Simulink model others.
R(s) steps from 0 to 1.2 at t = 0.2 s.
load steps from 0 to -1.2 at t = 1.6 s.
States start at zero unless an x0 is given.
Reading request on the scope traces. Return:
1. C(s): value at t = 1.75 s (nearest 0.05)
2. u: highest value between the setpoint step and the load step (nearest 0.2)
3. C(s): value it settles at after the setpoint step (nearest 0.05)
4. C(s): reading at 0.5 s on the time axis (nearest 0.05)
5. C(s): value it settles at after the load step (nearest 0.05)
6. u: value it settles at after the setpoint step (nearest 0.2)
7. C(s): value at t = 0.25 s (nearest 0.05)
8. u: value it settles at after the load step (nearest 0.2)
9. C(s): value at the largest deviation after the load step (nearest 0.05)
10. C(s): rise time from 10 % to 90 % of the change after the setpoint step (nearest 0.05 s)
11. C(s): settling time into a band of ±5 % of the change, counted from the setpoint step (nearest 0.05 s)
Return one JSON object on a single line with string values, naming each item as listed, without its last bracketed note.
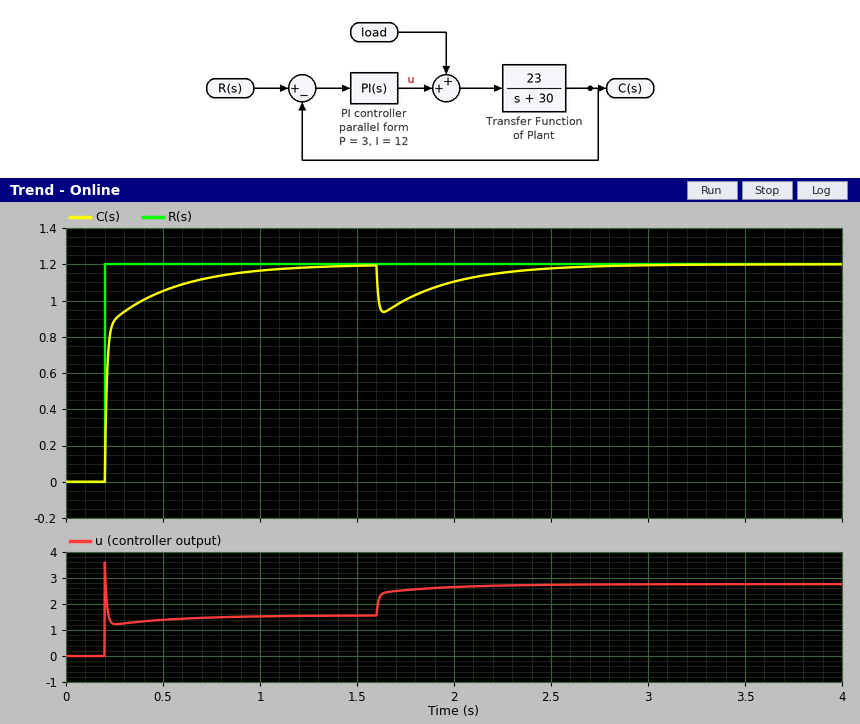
{"C(s): value at t = 1.75 s": "1.00", "u: highest value between the setpoint step and the load step": "3.6", "C(s): value it settles at after the setpoint step": "1.20", "C(s): reading at 0.5 s on the time axis": "1.05", "C(s): value it settles at after the load step": "1.20", "u: value it settles at after the setpoint step": "1.6", "C(s): value at t = 0.25 s": "0.90", "u: value it settles at after the load step": "2.8", "C(s): value at the largest deviation after the load step": "0.95", "C(s): rise time from 10 % to 90 % of the change after the setpoint step": "0.35 s", "C(s): settling time into a band of ±5 % of the change, counted from the setpoint step": "0.60 s"}
